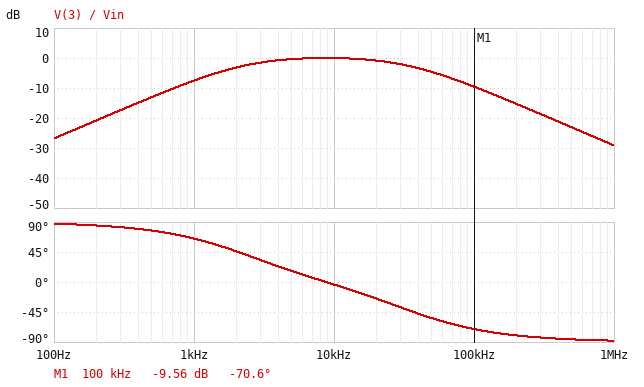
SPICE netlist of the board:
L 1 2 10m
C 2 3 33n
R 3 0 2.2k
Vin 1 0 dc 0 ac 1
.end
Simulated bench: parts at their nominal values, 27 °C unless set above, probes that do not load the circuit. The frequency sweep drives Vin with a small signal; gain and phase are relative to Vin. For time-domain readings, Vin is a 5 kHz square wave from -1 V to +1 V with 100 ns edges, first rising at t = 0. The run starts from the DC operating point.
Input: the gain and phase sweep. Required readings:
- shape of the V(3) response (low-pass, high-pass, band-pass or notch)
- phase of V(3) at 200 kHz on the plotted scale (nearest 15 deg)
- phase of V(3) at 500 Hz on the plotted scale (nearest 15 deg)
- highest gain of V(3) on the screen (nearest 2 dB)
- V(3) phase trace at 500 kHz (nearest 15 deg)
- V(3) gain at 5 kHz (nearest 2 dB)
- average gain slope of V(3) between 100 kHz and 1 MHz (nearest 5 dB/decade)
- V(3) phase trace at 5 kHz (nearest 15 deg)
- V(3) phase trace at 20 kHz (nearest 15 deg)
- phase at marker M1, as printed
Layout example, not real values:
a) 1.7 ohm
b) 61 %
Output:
a) band-pass
b) -75 deg
c) 75 deg
d) 0 dB
e) -90 deg
f) 0 dB
g) -20 dB/decade
h) 15 deg
i) -30 deg
j) -70.6 deg
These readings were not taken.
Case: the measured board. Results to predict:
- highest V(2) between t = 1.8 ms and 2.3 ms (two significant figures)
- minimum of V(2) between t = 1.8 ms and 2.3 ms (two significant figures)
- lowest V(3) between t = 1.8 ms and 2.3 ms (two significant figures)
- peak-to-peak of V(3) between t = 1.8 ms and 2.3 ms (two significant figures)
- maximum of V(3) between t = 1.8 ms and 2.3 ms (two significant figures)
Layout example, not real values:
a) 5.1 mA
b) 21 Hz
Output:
a) 1.1 V
b) -1.1 V
c) -1.4 V
d) 2.8 V
e) 1.4 V
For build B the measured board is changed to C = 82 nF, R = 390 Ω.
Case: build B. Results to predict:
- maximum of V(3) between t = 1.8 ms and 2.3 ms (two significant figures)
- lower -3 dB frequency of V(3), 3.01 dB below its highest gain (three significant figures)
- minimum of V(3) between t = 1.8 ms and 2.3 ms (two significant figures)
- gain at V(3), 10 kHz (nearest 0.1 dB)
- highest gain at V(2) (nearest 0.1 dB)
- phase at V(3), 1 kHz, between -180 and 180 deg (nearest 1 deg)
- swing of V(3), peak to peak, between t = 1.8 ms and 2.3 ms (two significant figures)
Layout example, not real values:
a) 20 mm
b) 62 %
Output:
a) 1.3 V
b) 3.26 kHz
c) -1.3 V
d) -3.5 dB
e) 2.9 dB
f) 78 deg
g) 2.6 V
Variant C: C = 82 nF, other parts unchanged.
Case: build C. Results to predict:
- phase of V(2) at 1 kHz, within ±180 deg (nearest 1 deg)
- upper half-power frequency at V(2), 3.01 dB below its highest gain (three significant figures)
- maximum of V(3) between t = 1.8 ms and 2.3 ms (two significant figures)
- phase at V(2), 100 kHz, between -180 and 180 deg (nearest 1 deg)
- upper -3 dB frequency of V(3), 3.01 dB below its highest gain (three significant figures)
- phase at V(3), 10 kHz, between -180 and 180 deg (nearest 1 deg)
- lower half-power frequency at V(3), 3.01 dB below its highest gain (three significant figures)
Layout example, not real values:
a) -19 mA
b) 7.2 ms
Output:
a) -1 deg
b) 34.5 kHz
c) 1.2 V
d) -71 deg
e) 35.9 kHz
f) -11 deg
g) 861 Hz
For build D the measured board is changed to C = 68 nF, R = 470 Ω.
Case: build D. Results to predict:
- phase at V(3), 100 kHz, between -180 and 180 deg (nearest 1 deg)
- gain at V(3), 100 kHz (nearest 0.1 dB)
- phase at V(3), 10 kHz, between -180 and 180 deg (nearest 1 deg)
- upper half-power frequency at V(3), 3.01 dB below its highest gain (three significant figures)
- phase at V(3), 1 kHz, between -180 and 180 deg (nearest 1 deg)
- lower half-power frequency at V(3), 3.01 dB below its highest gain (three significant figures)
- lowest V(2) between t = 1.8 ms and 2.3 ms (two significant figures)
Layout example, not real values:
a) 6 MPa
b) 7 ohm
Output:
a) -86 deg
b) -22.5 dB
c) -40 deg
d) 10.9 kHz
e) 78 deg
f) 3.42 kHz
g) -1.5 V
